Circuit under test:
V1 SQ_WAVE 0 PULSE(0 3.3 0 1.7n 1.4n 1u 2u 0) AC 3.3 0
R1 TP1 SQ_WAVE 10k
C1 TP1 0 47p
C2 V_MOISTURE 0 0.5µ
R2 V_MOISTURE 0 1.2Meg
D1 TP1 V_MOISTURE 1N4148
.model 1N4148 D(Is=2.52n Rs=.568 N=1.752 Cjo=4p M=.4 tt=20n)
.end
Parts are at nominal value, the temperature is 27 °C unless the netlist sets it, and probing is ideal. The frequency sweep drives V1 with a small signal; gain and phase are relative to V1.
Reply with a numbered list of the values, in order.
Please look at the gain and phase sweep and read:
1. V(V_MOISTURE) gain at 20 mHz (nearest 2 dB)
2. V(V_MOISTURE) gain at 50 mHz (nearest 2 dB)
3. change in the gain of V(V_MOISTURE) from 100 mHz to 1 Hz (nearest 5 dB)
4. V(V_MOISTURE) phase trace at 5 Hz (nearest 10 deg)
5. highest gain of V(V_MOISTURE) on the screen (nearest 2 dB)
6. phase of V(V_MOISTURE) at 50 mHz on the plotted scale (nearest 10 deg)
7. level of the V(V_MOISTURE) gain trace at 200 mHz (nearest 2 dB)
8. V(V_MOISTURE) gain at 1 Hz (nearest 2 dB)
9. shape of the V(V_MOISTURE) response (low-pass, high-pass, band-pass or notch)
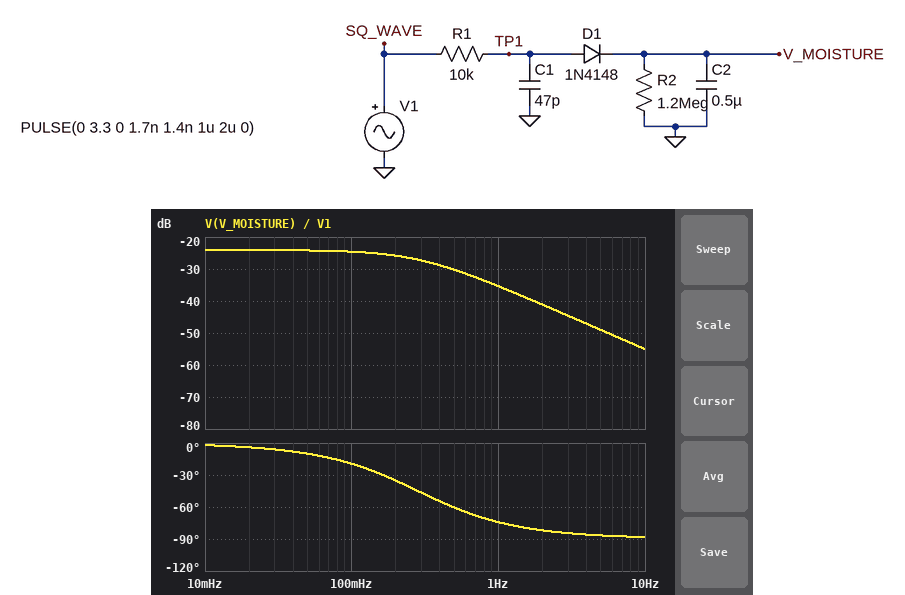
1. -24 dB
2. -24 dB
3. -10 dB
4. -90 deg
5. -24 dB
6. -10 deg
7. -26 dB
8. -36 dB
9. low-pass
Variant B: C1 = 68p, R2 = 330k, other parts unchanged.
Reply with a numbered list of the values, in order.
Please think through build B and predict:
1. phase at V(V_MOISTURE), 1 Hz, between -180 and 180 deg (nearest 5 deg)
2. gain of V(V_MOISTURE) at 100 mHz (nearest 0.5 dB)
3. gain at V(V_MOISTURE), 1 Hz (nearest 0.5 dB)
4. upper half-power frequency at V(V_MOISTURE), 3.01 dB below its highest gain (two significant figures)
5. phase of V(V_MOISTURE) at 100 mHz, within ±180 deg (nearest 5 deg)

1. -45 deg
2. -35.0 dB
3. -38.0 dB
4. 980 mHz
5. -5 deg
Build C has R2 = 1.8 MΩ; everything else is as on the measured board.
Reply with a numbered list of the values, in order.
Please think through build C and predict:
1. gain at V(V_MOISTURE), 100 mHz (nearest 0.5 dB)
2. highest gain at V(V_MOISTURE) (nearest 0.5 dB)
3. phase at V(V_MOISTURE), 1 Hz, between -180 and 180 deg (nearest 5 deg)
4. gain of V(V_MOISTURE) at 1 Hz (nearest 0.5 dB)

1. -22.0 dB
2. -21.0 dB
3. -80 deg
4. -35.0 dB
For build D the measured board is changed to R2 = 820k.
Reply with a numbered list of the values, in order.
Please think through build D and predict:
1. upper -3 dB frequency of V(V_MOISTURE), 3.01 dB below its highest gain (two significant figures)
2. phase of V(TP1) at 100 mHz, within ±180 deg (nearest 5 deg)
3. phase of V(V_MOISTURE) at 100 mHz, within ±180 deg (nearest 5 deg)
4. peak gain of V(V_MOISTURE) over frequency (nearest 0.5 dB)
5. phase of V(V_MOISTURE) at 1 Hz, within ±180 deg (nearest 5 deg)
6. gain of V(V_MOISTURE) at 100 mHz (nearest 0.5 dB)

1. 410 mHz
2. 0 deg
3. -15 deg
4. -27.0 dB
5. -70 deg
6. -27.5 dB
